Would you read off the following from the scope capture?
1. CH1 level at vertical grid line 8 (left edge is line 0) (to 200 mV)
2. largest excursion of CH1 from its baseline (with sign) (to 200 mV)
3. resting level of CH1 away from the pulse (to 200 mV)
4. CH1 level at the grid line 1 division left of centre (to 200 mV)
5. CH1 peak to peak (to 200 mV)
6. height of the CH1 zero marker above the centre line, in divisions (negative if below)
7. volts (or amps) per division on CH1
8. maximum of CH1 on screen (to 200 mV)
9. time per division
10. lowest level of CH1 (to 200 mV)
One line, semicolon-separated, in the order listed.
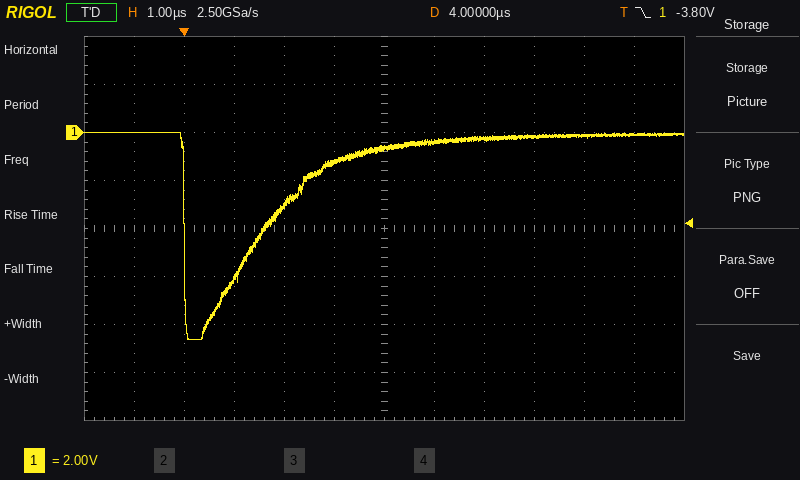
-200 mV; -8.4 V; -200 mV; -1.2 V; 8.6 V; +2.0 div; 2 V; 0.0 V; 1 µs; -8.6 V
